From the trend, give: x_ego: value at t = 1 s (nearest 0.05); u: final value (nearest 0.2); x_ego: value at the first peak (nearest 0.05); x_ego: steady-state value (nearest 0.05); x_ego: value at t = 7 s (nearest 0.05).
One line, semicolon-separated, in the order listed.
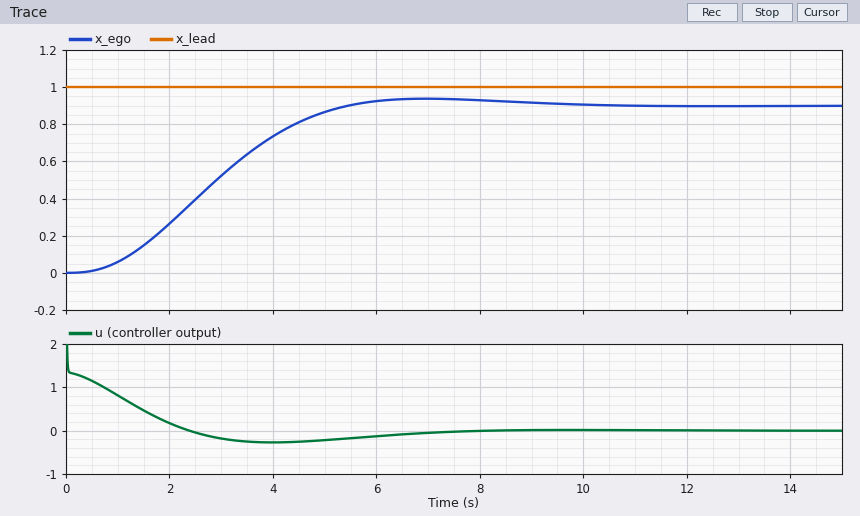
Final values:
0.05; 0.0; 0.95; 0.90; 0.95
